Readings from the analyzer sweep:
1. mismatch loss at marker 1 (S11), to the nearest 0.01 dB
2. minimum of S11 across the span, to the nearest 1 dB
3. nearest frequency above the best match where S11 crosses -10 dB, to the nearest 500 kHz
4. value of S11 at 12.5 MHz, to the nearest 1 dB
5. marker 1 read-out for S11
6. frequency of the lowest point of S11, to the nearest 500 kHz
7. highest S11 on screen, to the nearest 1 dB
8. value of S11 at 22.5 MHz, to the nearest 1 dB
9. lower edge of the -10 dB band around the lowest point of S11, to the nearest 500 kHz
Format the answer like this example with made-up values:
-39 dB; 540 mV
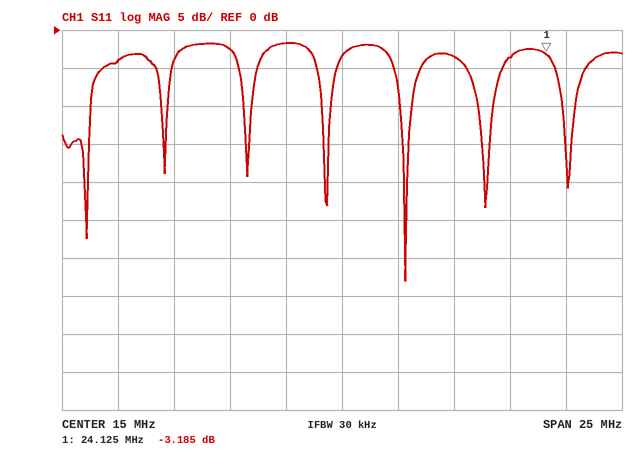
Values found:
2.84 dB; -33 dB; 18.0 MHz; -2 dB; -3.185 dB; 18.0 MHz; -2 dB; -4 dB; 17.5 MHz
